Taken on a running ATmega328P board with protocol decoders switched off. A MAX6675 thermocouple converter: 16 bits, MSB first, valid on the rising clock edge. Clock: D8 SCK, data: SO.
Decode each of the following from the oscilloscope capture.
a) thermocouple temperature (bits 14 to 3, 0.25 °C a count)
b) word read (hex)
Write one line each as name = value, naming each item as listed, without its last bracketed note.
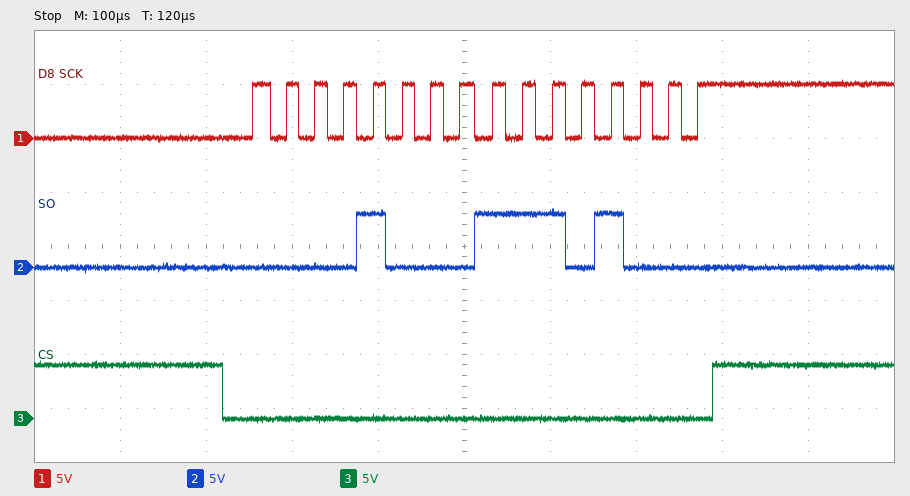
thermocouple temperature = 71.25 °C
word read = 0x08E8
